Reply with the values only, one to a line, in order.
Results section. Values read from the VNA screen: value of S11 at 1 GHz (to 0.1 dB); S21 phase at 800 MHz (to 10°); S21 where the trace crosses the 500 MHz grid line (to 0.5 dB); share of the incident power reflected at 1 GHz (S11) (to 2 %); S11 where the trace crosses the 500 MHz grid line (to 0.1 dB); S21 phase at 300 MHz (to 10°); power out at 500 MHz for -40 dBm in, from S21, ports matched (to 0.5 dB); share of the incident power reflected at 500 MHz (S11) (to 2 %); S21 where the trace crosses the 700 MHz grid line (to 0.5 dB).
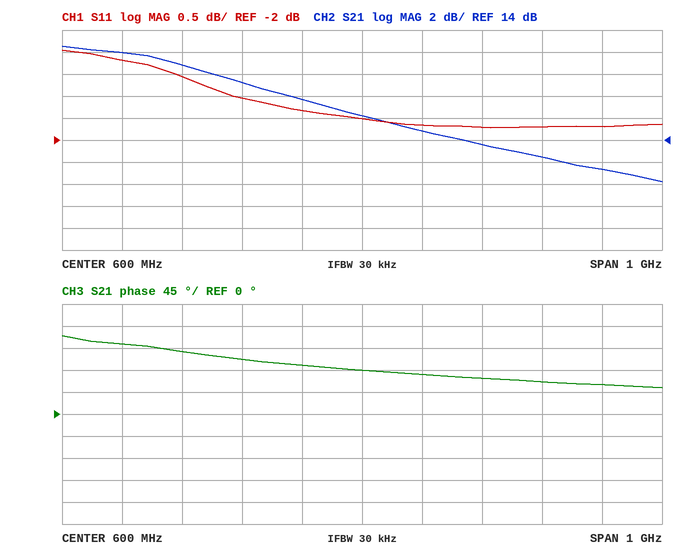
-1.7 dB
70°
17.5 dB
68 %
-1.3 dB
130°
-22.5 dBm
74 %
15.0 dB
